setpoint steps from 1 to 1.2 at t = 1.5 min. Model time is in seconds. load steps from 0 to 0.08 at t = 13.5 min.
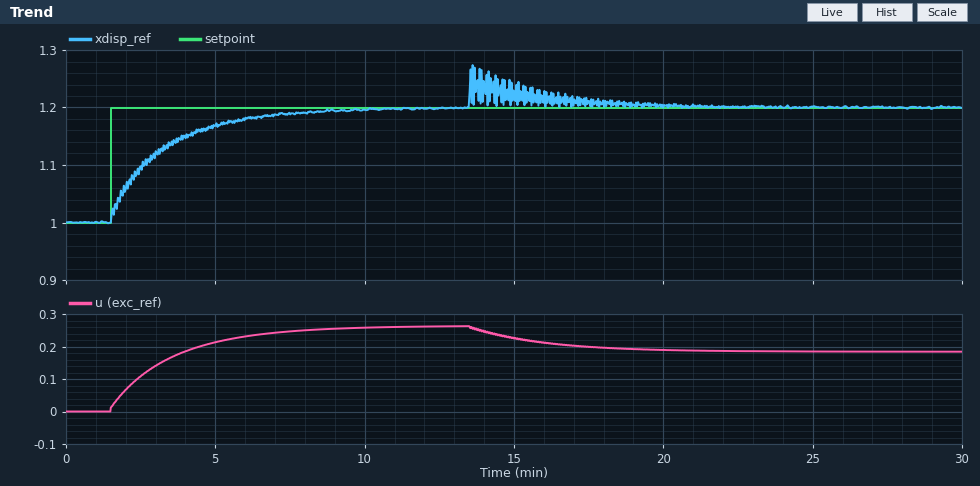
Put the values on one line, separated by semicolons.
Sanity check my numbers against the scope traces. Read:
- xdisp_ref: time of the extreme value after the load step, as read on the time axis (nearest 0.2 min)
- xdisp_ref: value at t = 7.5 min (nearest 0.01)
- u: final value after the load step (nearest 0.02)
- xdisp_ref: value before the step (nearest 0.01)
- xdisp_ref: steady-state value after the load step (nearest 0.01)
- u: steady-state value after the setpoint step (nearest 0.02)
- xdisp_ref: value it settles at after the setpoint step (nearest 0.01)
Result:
13.6 min; 1.19; 0.18; 1.00; 1.20; 0.26; 1.20
